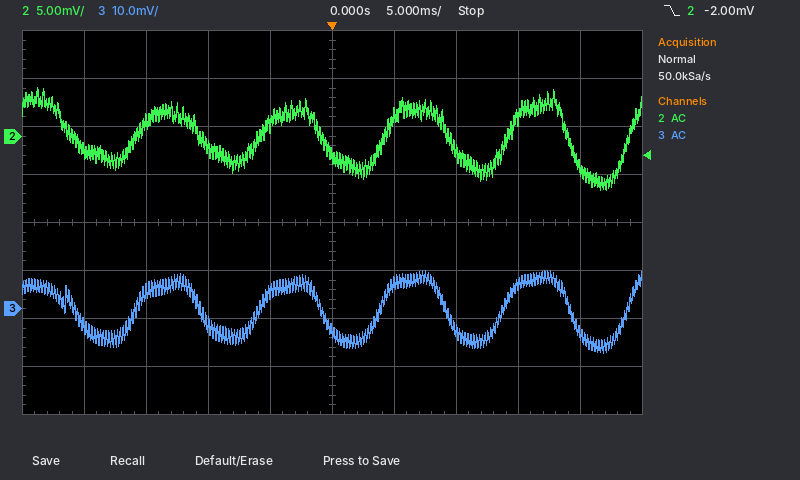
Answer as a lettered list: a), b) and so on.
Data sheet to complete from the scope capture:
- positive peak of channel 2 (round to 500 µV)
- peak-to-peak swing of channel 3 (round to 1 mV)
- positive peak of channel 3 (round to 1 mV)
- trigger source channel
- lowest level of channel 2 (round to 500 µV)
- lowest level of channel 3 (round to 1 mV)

a) 5.0 mV
b) 17 mV
c) 8 mV
d) channel 2
e) -5.5 mV
f) -9 mV
